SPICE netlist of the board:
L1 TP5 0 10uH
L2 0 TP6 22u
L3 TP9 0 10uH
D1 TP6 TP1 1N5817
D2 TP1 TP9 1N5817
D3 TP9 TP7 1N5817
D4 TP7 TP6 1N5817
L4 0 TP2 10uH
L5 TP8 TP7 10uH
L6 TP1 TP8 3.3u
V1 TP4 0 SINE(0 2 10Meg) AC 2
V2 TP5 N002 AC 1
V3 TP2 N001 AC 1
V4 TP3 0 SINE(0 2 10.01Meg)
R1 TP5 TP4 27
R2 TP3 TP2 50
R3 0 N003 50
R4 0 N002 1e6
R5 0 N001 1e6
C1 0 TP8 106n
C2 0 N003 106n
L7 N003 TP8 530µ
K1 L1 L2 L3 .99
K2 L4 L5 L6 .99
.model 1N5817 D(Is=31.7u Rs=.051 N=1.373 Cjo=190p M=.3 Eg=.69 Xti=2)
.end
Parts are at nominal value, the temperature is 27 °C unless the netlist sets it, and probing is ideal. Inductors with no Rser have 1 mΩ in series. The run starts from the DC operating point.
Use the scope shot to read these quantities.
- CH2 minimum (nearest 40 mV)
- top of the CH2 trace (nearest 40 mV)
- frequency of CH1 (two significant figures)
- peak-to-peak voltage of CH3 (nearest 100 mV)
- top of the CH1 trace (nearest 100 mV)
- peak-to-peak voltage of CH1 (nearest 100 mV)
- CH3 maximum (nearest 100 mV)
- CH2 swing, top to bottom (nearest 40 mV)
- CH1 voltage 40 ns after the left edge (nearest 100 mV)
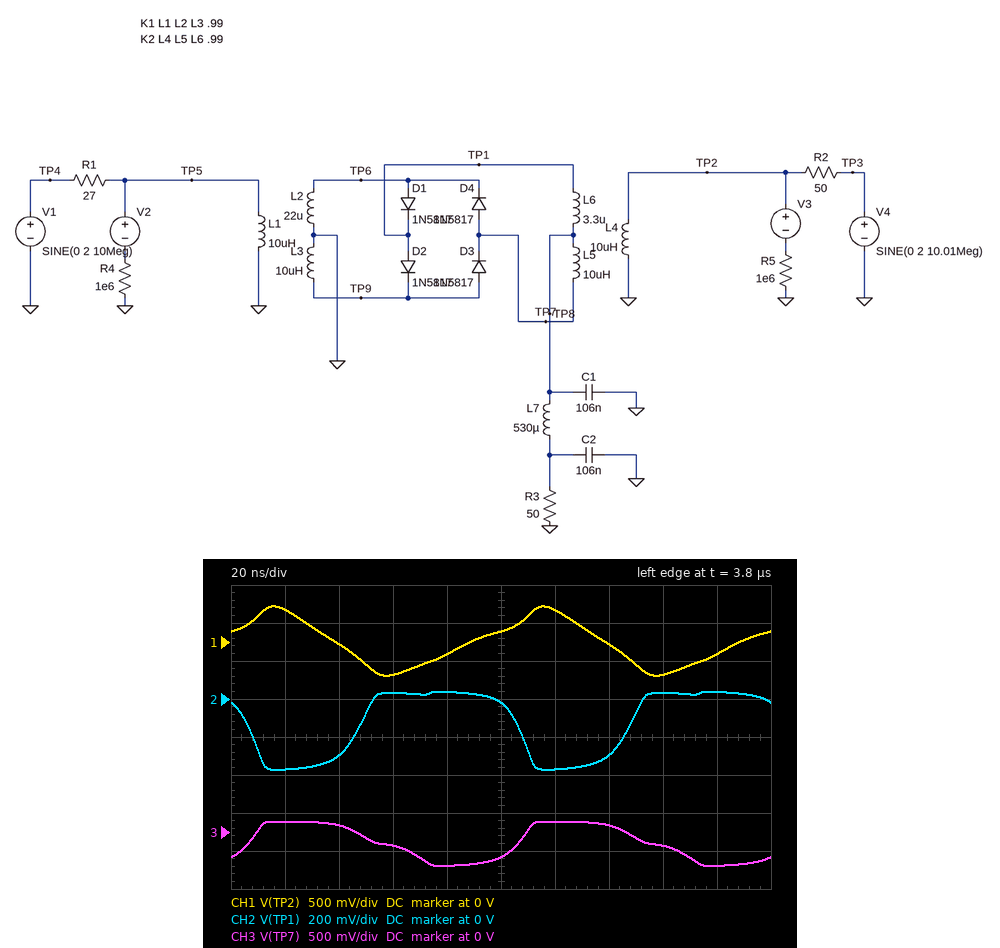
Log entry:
-360 mV
40 mV
10 MHz
600 mV
500 mV
900 mV
100 mV
400 mV
0 V
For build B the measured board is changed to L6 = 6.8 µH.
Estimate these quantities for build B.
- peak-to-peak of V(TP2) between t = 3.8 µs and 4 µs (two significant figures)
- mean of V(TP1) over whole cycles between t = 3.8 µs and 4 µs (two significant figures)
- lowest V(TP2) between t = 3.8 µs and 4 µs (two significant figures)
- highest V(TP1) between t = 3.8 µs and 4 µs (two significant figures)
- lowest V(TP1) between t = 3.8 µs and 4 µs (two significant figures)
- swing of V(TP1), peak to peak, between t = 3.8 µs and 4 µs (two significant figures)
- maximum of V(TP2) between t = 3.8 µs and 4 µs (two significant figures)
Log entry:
720 mV
-150 mV
-360 mV
56 mV
-430 mV
480 mV
360 mV
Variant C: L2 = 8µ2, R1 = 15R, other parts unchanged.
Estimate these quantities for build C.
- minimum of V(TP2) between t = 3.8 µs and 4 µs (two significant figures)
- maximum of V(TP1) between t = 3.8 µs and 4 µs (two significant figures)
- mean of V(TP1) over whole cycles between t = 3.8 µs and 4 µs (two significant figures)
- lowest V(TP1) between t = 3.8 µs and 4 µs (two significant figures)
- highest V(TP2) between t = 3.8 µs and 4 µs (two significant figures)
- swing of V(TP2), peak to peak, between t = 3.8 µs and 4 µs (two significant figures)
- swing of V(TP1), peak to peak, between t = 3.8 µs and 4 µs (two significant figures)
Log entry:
-480 mV
100 mV
-140 mV
-400 mV
460 mV
940 mV
500 mV
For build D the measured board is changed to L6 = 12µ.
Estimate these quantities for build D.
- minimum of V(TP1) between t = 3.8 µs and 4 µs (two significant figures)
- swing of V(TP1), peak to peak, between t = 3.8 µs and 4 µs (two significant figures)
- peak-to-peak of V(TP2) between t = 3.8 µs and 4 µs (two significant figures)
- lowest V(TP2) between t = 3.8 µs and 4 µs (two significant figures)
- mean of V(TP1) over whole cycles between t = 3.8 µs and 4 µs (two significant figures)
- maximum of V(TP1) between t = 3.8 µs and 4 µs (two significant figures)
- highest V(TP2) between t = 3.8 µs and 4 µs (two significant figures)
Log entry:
-470 mV
540 mV
600 mV
-300 mV
-170 mV
71 mV
290 mV
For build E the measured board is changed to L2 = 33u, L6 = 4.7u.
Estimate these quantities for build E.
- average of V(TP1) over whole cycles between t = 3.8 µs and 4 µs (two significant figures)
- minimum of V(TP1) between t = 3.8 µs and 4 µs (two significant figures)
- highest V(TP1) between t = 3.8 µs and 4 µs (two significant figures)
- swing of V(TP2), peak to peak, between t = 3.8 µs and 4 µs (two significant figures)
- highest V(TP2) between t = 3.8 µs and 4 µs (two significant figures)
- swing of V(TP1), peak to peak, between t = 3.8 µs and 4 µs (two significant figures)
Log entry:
-130 mV
-390 mV
57 mV
810 mV
410 mV
450 mV
